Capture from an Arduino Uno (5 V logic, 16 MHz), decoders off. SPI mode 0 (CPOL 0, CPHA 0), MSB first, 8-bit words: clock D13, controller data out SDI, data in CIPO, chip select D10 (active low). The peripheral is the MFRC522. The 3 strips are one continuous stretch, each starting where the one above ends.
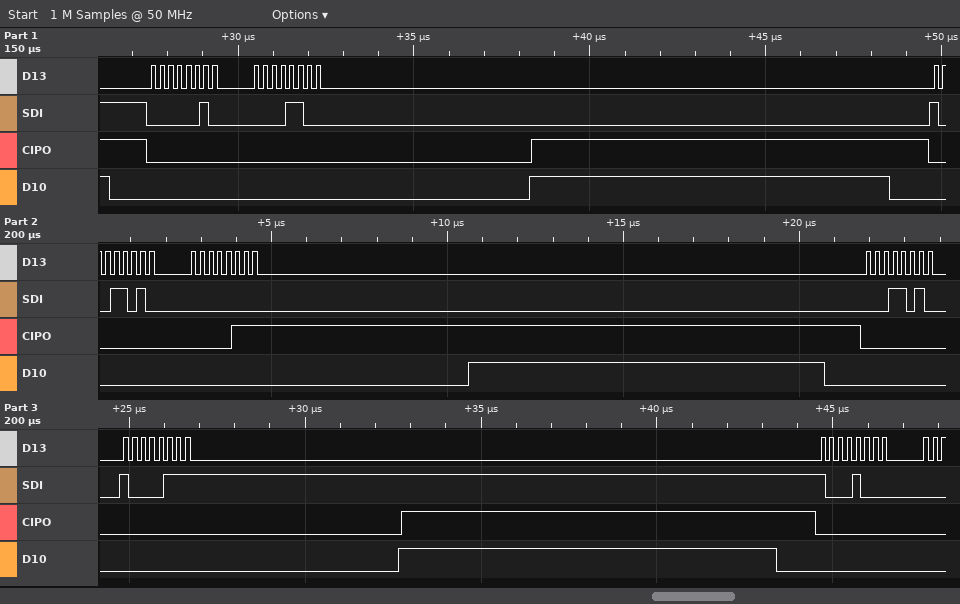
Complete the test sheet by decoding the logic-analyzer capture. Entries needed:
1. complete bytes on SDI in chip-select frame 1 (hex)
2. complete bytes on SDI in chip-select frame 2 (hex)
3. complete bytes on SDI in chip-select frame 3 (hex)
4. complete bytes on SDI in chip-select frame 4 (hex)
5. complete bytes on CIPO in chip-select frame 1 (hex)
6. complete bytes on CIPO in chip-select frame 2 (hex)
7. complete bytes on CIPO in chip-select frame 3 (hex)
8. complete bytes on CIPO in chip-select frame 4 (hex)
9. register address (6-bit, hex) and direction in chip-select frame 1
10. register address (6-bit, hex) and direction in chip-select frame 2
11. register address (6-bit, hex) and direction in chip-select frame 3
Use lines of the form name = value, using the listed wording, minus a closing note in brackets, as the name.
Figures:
complete bytes on SDI in chip-select frame 1 = 02 0C
complete bytes on SDI in chip-select frame 2 = 9A 00
complete bytes on SDI in chip-select frame 3 = 1A 87
complete bytes on SDI in chip-select frame 4 = 88
complete bytes on CIPO in chip-select frame 1 = 00 00
complete bytes on CIPO in chip-select frame 2 = 00 07
complete bytes on CIPO in chip-select frame 3 = 00 00
complete bytes on CIPO in chip-select frame 4 = 00
register address (6-bit, hex) and direction in chip-select frame 1 = 0x01 write
register address (6-bit, hex) and direction in chip-select frame 2 = 0x0D read
register address (6-bit, hex) and direction in chip-select frame 3 = 0x0D write
